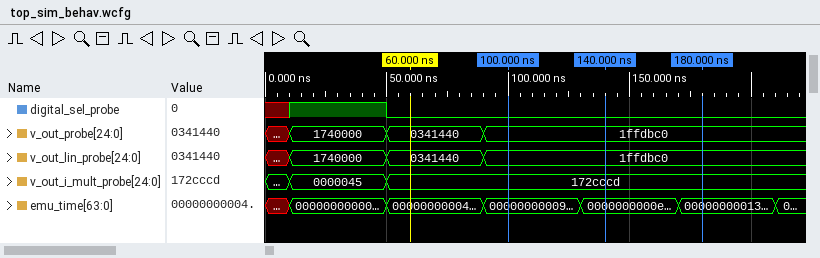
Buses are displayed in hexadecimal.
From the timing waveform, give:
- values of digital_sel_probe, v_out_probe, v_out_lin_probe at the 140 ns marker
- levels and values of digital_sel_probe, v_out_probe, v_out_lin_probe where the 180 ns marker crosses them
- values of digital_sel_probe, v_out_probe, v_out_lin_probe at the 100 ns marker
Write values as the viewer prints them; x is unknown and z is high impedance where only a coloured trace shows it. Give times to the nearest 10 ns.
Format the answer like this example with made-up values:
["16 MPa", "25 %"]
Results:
["digital_sel_probe=0, v_out_probe=1ffdbc0, v_out_lin_probe=1ffdbc0", "digital_sel_probe=0, v_out_probe=1ffdbc0, v_out_lin_probe=1ffdbc0", "digital_sel_probe=0, v_out_probe=1ffdbc0, v_out_lin_probe=1ffdbc0"]
